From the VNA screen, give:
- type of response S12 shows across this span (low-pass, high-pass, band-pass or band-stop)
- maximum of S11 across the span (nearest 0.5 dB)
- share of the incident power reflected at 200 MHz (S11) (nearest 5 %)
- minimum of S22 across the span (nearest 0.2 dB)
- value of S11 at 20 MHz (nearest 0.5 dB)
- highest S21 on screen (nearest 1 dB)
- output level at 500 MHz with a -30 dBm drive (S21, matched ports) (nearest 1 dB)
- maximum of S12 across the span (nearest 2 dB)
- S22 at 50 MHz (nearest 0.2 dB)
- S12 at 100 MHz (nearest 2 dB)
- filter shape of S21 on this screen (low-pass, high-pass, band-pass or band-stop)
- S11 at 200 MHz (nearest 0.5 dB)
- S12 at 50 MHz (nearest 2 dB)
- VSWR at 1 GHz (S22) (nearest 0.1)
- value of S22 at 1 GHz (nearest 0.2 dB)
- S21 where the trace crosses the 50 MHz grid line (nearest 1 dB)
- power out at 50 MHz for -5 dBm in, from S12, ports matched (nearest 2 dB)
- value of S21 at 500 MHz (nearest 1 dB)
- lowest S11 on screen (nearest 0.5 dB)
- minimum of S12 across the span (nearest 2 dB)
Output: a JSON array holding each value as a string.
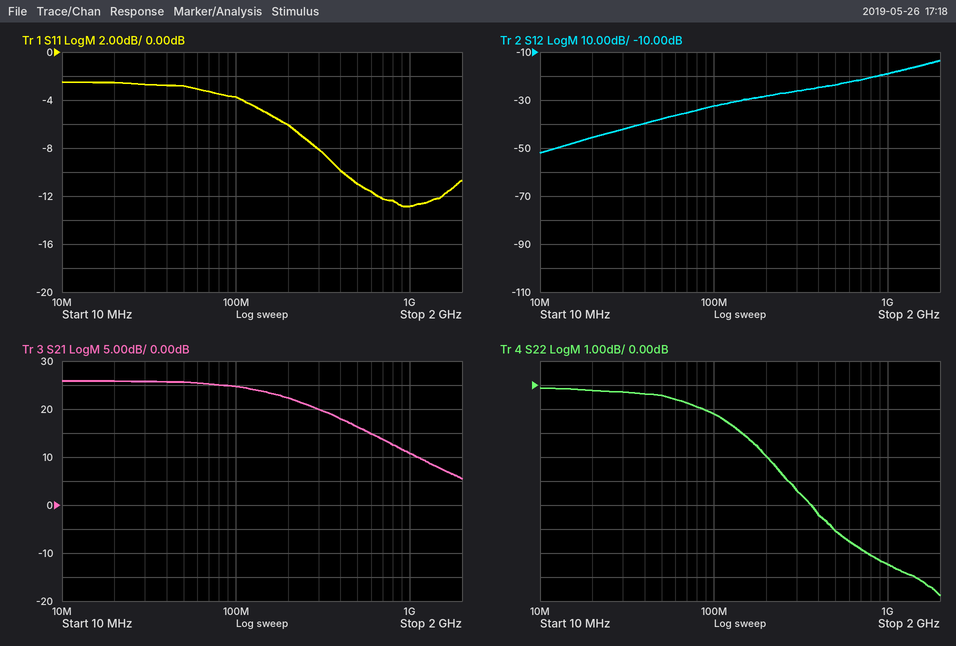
["high-pass", "-2.5 dB", "25 %", "-8.8 dB", "-2.5 dB", "26 dB", "-14 dBm", "-14 dB", "-0.4 dB", "-32 dB", "low-pass", "-6.0 dB", "-38 dB", "2.5", "-7.4 dB", "26 dB", "-42 dBm", "16 dB", "-13.0 dB", "-52 dB"]
